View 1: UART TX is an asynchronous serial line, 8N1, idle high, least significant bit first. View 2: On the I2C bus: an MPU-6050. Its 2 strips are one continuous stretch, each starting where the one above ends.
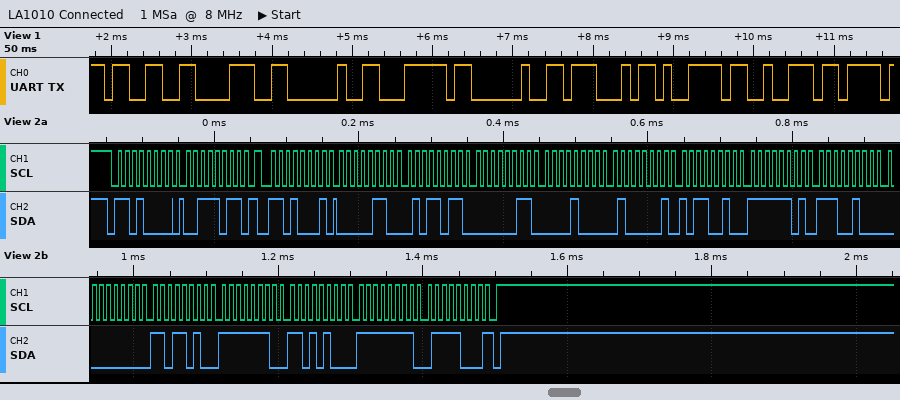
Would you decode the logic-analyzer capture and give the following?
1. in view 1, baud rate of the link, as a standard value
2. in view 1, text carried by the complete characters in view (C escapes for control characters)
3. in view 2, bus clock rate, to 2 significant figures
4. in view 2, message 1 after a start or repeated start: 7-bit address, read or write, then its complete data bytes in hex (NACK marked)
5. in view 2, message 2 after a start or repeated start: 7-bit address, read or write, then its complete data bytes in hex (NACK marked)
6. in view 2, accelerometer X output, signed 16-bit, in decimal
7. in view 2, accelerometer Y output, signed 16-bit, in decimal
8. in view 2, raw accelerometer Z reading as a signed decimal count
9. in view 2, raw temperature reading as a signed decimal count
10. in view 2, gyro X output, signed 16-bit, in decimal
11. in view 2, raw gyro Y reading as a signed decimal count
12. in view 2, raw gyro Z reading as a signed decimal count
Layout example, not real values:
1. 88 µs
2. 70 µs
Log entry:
1. 9600 baud
2. "38 | Gyr"
3. 100 kHz
4. 0x68 write: 3B
5. 0x68 read: 06 5B 03 08 41 B2 FD E4 00 DA FE D4 FF 78 NACK
6. 1627
7. 776
8. 16818
9. -540
10. 218
11. -300
12. -136
